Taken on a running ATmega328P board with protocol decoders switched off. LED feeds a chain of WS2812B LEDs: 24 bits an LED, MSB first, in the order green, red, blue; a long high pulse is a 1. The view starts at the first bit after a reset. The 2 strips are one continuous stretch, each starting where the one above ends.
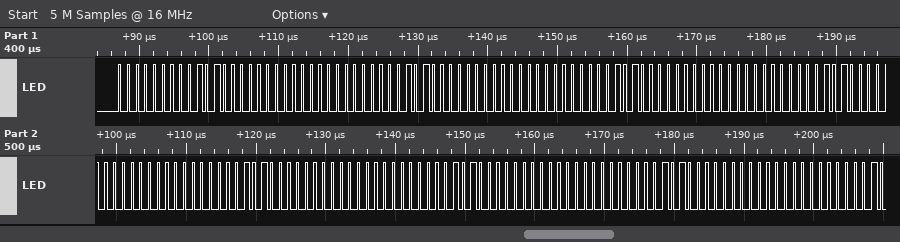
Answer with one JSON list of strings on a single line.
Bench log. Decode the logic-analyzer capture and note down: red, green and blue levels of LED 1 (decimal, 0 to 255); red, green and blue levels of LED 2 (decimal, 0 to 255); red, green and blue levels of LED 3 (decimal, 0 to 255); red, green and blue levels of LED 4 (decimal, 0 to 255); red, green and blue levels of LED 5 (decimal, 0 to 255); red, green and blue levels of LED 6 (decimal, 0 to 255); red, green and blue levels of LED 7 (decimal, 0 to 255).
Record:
["80, 0, 0", "80, 0, 0", "80, 0, 0", "80, 0, 0", "80, 0, 0", "80, 0, 0", "80, 0, 0"]
